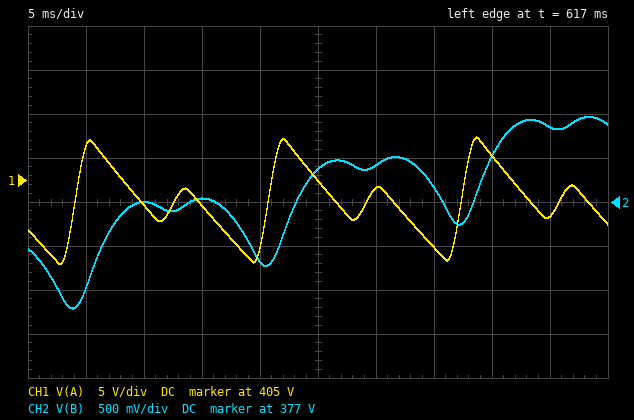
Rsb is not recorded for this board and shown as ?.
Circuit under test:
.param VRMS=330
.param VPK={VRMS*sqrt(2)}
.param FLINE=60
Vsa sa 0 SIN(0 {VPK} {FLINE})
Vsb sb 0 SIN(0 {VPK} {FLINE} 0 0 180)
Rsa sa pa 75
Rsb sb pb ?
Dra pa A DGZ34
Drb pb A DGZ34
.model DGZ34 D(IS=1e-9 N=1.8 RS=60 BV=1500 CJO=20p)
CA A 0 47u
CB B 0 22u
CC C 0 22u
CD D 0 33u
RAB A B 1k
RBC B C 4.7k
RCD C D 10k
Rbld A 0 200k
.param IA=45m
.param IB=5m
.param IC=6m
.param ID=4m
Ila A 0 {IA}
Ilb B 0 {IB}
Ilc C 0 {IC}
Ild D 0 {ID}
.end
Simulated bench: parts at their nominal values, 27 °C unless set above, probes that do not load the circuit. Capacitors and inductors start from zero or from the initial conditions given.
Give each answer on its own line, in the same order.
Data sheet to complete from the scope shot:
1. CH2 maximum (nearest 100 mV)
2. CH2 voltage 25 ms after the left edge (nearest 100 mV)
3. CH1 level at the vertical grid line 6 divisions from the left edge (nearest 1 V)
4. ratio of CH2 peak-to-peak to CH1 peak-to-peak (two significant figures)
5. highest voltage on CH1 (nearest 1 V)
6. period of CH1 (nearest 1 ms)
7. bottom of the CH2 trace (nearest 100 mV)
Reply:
378.0 V
377.4 V
404 V
0.15
410 V
17 ms
375.8 V
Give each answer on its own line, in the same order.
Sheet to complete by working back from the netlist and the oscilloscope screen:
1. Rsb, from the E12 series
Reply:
270 Ω
